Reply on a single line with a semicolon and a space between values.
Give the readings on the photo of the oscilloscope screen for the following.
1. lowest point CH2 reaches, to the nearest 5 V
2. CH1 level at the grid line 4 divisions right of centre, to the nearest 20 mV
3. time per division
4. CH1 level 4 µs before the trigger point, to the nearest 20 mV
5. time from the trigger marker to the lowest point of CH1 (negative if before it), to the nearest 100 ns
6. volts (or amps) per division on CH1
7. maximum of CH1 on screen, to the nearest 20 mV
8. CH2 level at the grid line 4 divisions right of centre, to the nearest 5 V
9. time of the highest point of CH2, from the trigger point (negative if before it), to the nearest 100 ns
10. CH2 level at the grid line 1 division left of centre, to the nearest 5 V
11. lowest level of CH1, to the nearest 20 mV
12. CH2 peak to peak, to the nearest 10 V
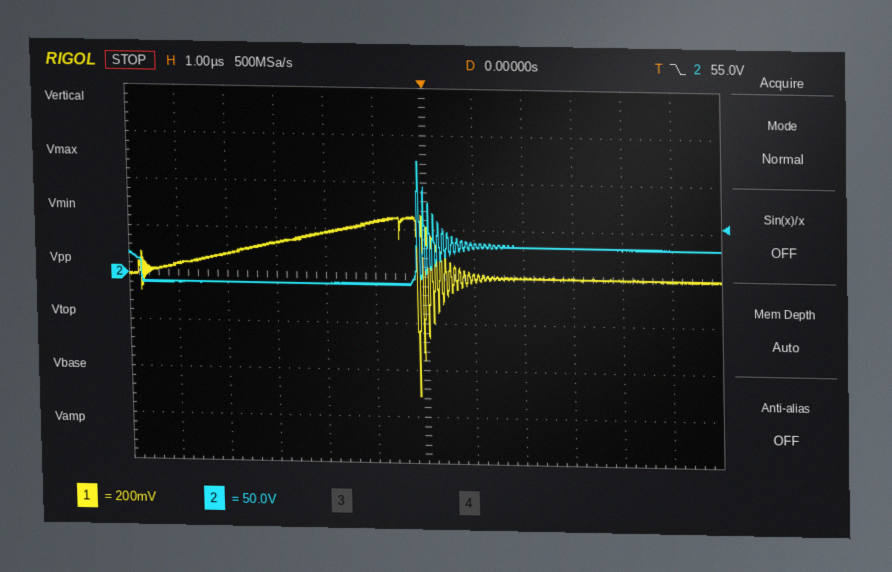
-10 V; 0 mV; 1 µs; 80 mV; -100 ns; 200 mV; 260 mV; 35 V; -100 ns; -10 V; -500 mV; 130 V
